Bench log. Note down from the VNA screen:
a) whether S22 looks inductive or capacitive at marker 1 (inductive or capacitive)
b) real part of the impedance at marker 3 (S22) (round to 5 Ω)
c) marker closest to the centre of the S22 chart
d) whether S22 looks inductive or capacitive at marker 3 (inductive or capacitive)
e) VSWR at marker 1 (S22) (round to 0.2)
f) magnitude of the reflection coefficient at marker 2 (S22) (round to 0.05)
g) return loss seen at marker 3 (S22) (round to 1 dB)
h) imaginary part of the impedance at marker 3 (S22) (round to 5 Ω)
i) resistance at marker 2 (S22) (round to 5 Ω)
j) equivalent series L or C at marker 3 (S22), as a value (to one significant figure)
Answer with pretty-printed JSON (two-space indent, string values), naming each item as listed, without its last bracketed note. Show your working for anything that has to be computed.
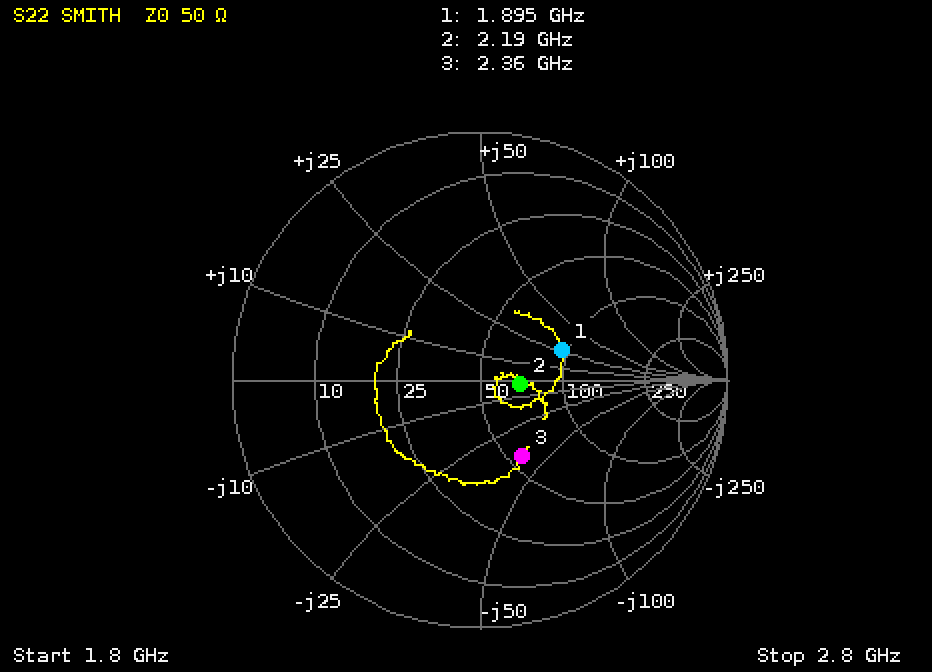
{
  "whether S22 looks inductive or capacitive at marker 1": "inductive",
  "real part of the impedance at marker 3 (S22)": "55 Ω",
  "marker closest to the centre of the S22 chart": "marker 2",
  "whether S22 looks inductive or capacitive at marker 3": "capacitive",
  "VSWR at marker 1 (S22)": "2.0",
  "magnitude of the reflection coefficient at marker 2 (S22)": "0.15",
  "return loss seen at marker 3 (S22)": "9 dB",
  "imaginary part of the impedance at marker 3 (S22)": "-40 Ω",
  "resistance at marker 2 (S22)": "70 Ω",
  "equivalent series L or C at marker 3 (S22), as a value": "C = 1/(2π × 2.36 GHz × 40 Ω) ≈ 2 pF"
}
